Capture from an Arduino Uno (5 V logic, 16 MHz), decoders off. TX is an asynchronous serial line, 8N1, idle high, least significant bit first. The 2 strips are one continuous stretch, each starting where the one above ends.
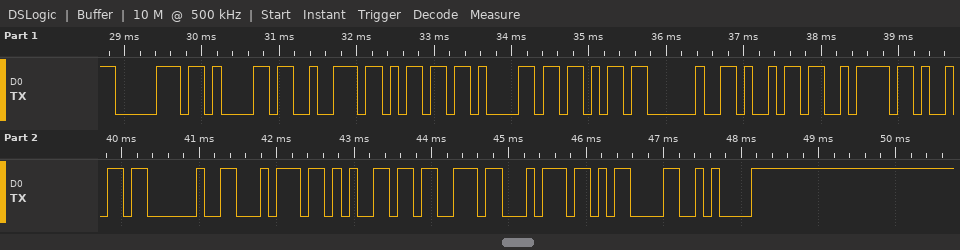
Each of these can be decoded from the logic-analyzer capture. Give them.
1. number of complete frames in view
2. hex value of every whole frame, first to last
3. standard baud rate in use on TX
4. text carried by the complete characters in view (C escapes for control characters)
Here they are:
17
70 61 72 6D 61 6B 20 69 7A 69 20 74 65 73 74 0D 0A
9600 baud
"parmak izi test\r\n"
